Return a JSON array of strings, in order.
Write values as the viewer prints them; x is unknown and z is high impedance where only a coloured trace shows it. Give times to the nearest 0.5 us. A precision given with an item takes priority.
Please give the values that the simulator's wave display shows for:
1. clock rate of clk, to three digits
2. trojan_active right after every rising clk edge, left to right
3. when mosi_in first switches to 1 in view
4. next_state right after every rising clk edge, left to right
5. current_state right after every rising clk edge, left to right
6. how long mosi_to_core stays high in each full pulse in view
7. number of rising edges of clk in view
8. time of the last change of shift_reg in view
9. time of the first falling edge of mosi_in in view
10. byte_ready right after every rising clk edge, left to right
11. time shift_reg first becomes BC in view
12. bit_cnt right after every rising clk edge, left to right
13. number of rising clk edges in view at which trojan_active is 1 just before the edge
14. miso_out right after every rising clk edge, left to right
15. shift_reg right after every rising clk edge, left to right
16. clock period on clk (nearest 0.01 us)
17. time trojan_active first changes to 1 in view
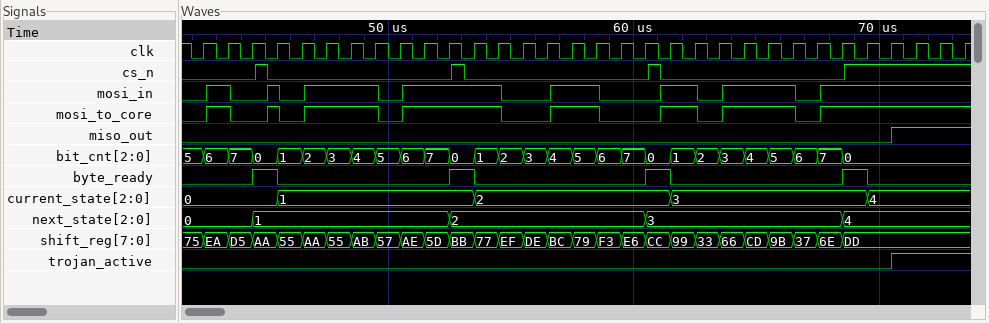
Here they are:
["1.00 MHz", "0 0 0 0 0 0 0 0 0 0 0 0 0 0 0 0 0 0 0 0 0 0 0 0 0 0 0 0 1 1 1 1", "42.5 us", "0, 0, 1, 1, 1, 1, 1, 1, 1, 1, 2, 2, 2, 2, 2, 2, 2, 2, 3, 3, 3, 3, 3, 3, 3, 3, 4, 4, 4, 4, 4, 4", "0, 0, 0, 1, 1, 1, 1, 1, 1, 1, 1, 2, 2, 2, 2, 2, 2, 2, 2, 3, 3, 3, 3, 3, 3, 3, 3, 4, 4, 4, 4, 4", "1 us, 0.5 us, 3 us, 4 us, 2 us, 1.5 us, 3 us", "32", "68.5 us", "43.5 us", "0 0 1 0 0 0 0 0 0 0 1 0 0 0 0 0 0 0 1 0 0 0 0 0 0 0 1 0 0 0 0 0", "56.5 us", "6, 7, 0, 1, 2, 3, 4, 5, 6, 7, 0, 1, 2, 3, 4, 5, 6, 7, 0, 1, 2, 3, 4, 5, 6, 7, 0, 0, 0, 0, 0, 0", "3", "0 0 0 0 0 0 0 0 0 0 0 0 0 0 0 0 0 0 0 0 0 0 0 0 0 0 0 0 1 1 1 1", "EA, D5, AA, 55, AA, 55, AB, 57, AE, 5D, BB, 77, EF, DE, BC, 79, F3, E6, CC, 99, 33, 66, CD, 9B, 37, 6E, DD, DD, DD, DD, DD, DD", "1 us", "70.5 us"]
